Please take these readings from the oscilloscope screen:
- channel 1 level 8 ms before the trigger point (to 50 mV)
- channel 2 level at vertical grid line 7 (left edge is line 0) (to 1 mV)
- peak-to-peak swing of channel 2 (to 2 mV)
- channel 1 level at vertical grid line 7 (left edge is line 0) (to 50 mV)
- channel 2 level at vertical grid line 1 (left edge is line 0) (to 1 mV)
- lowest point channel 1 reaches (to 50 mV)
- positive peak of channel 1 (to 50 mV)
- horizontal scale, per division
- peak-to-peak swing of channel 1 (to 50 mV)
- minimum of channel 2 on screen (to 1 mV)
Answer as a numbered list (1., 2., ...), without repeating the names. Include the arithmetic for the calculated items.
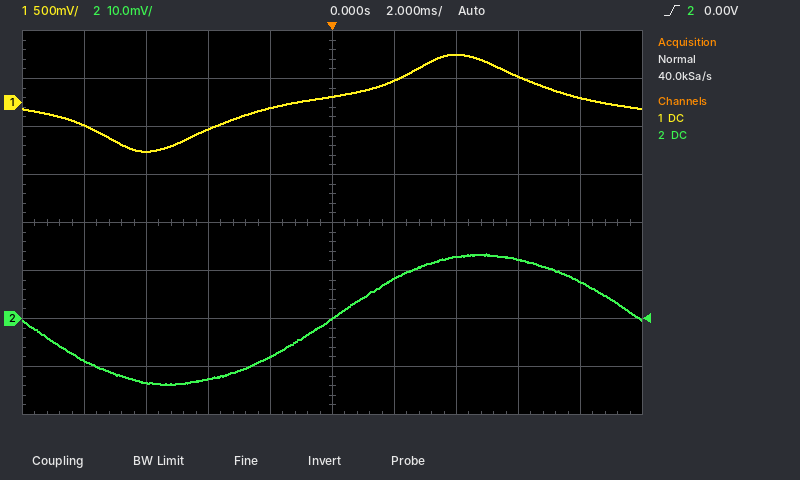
1. -250 mV
2. 13 mV
3. 28 mV
4. 500 mV
5. -9 mV
6. -500 mV
7. 500 mV
8. 2 ms
9. 500 mV − (-500 mV) = 1.00 V
10. -14 mV
